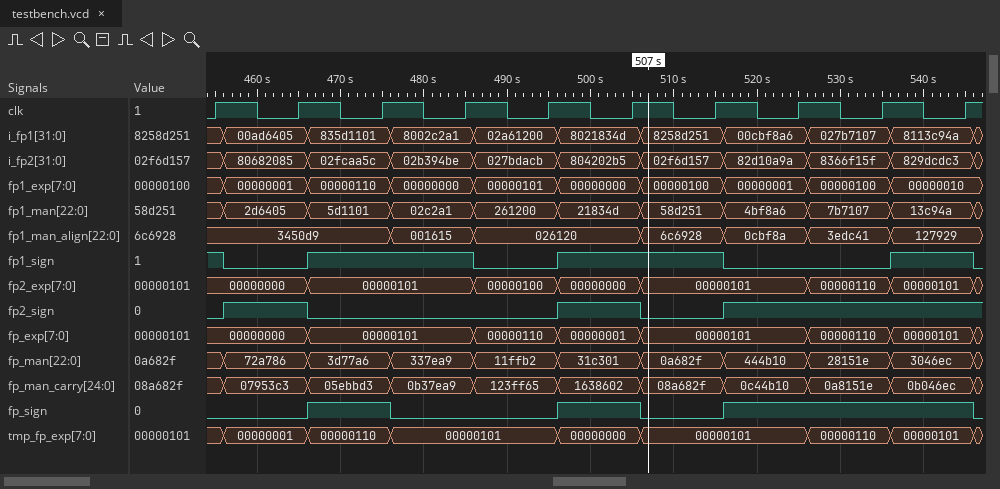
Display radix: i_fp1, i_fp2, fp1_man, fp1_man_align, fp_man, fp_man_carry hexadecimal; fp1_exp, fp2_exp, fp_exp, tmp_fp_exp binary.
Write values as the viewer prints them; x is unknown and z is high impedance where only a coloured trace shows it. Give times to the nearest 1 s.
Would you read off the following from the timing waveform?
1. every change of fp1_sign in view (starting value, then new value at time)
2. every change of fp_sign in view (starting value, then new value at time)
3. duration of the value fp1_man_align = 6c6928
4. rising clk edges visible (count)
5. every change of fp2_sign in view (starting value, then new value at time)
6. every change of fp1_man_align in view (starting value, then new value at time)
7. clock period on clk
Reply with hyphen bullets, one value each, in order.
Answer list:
- 1, 0 at 456 s, 1 at 466 s, 0 at 486 s, 1 at 496 s, 0 at 516 s, 1 at 536 s, 0 at 546 s
- 0, 1 at 466 s, 0 at 476 s, 1 at 496 s, 0 at 506 s, 1 at 516 s, 0 at 546 s
- 10 s
- 10
- 0, 1 at 456 s, 0 at 466 s, 1 at 496 s, 0 at 506 s, 1 at 516 s
- 3450d9, 001615 at 476 s, 026120 at 486 s, 6c6928 at 506 s, 0cbf8a at 516 s, 3edc41 at 526 s, 127929 at 536 s
- 10 s
